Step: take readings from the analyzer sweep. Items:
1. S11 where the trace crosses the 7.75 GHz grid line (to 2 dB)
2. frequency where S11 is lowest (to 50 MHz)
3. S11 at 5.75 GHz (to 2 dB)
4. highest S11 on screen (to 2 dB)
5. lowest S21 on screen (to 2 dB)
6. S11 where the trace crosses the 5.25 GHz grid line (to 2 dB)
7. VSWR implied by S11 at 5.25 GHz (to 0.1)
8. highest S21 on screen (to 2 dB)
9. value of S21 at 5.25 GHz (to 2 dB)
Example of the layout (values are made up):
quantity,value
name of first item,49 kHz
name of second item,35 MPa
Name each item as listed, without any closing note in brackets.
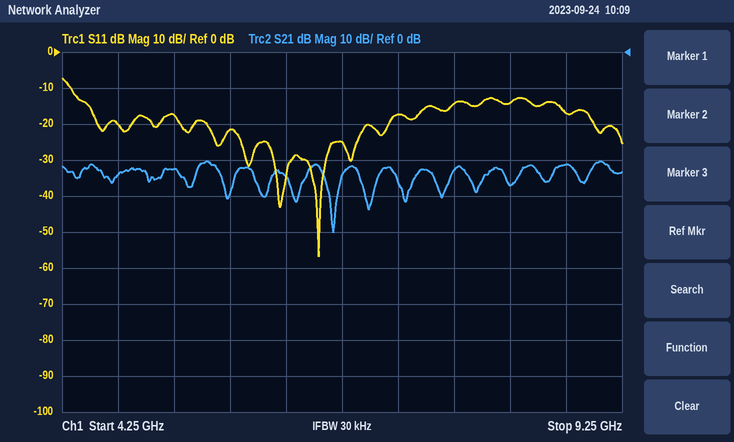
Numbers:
quantity,value
S11 where the trace crosses the 7.75 GHz grid line,-14 dB
frequency where S11 is lowest,6.55 GHz
S11 at 5.75 GHz,-22 dB
highest S11 on screen,-8 dB
lowest S21 on screen,-50 dB
S11 where the trace crosses the 5.25 GHz grid line,-18 dB
VSWR implied by S11 at 5.25 GHz,1.3
highest S21 on screen,-30 dB
value of S21 at 5.25 GHz,-32 dB
